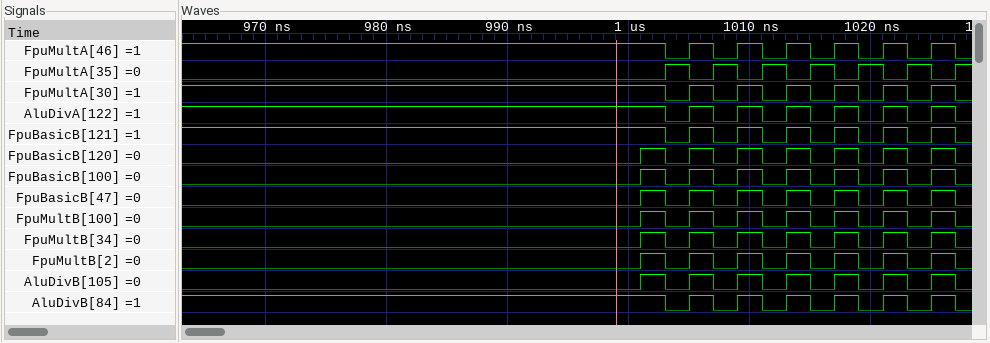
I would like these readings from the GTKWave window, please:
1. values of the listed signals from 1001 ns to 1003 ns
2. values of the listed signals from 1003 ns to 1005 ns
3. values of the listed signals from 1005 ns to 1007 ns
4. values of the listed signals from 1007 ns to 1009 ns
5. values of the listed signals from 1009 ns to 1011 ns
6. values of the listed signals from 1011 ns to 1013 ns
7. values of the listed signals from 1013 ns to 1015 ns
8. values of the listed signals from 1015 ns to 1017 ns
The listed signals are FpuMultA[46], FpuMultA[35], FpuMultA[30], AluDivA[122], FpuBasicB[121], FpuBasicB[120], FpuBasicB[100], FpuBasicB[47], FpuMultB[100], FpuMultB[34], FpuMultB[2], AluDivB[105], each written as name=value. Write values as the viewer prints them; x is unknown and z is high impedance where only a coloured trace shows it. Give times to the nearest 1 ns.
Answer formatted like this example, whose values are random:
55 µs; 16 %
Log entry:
FpuMultA[46]=1, FpuMultA[35]=0, FpuMultA[30]=1, AluDivA[122]=1, FpuBasicB[121]=1, FpuBasicB[120]=1, FpuBasicB[100]=1, FpuBasicB[47]=1, FpuMultB[100]=1, FpuMultB[34]=1, FpuMultB[2]=1, AluDivB[105]=1; FpuMultA[46]=0, FpuMultA[35]=1, FpuMultA[30]=0, AluDivA[122]=0, FpuBasicB[121]=0, FpuBasicB[120]=0, FpuBasicB[100]=0, FpuBasicB[47]=0, FpuMultB[100]=0, FpuMultB[34]=0, FpuMultB[2]=0, AluDivB[105]=0; FpuMultA[46]=1, FpuMultA[35]=0, FpuMultA[30]=1, AluDivA[122]=1, FpuBasicB[121]=1, FpuBasicB[120]=1, FpuBasicB[100]=1, FpuBasicB[47]=1, FpuMultB[100]=1, FpuMultB[34]=1, FpuMultB[2]=1, AluDivB[105]=1; FpuMultA[46]=0, FpuMultA[35]=1, FpuMultA[30]=0, AluDivA[122]=0, FpuBasicB[121]=0, FpuBasicB[120]=0, FpuBasicB[100]=0, FpuBasicB[47]=0, FpuMultB[100]=0, FpuMultB[34]=0, FpuMultB[2]=0, AluDivB[105]=0; FpuMultA[46]=1, FpuMultA[35]=0, FpuMultA[30]=1, AluDivA[122]=1, FpuBasicB[121]=1, FpuBasicB[120]=1, FpuBasicB[100]=1, FpuBasicB[47]=1, FpuMultB[100]=1, FpuMultB[34]=1, FpuMultB[2]=1, AluDivB[105]=1; FpuMultA[46]=0, FpuMultA[35]=1, FpuMultA[30]=0, AluDivA[122]=0, FpuBasicB[121]=0, FpuBasicB[120]=0, FpuBasicB[100]=0, FpuBasicB[47]=0, FpuMultB[100]=0, FpuMultB[34]=0, FpuMultB[2]=0, AluDivB[105]=0; FpuMultA[46]=1, FpuMultA[35]=0, FpuMultA[30]=1, AluDivA[122]=1, FpuBasicB[121]=1, FpuBasicB[120]=1, FpuBasicB[100]=1, FpuBasicB[47]=1, FpuMultB[100]=1, FpuMultB[34]=1, FpuMultB[2]=1, AluDivB[105]=1; FpuMultA[46]=0, FpuMultA[35]=1, FpuMultA[30]=0, AluDivA[122]=0, FpuBasicB[121]=0, FpuBasicB[120]=0, FpuBasicB[100]=0, FpuBasicB[47]=0, FpuMultB[100]=0, FpuMultB[34]=0, FpuMultB[2]=0, AluDivB[105]=0
